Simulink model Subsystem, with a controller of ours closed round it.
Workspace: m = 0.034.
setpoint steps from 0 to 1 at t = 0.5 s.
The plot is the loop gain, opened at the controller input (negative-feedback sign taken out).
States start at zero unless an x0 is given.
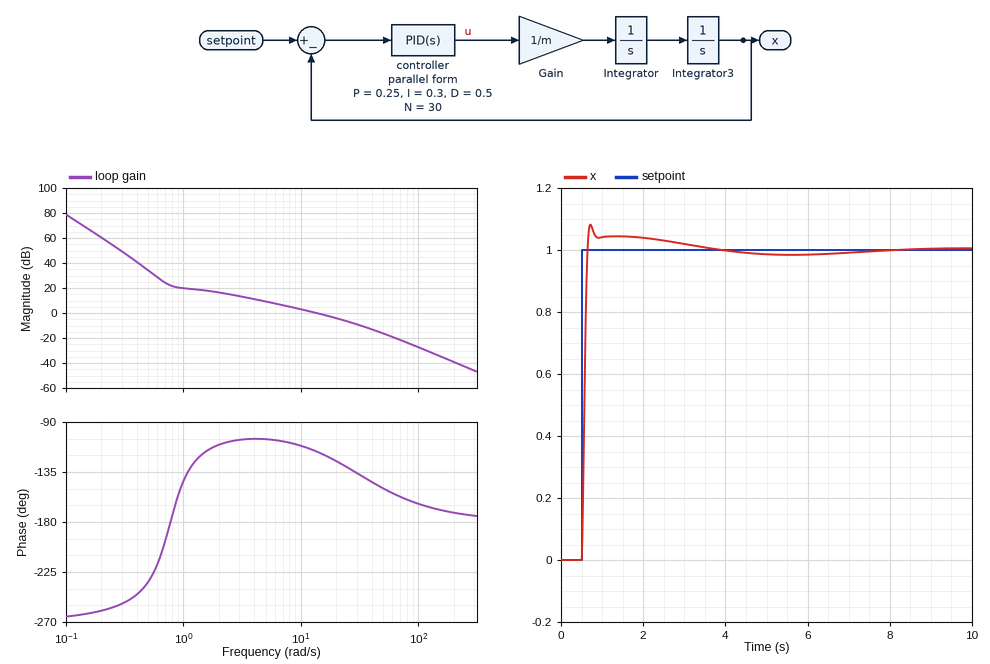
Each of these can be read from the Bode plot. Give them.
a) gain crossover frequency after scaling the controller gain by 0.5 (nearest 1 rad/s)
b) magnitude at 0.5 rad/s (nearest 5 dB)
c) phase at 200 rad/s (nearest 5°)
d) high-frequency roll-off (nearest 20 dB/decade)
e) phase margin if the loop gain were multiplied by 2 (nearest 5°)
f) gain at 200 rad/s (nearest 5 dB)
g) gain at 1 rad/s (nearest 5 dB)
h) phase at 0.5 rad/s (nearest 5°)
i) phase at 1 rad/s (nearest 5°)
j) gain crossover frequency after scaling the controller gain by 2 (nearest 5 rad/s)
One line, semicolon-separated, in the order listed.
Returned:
7 rad/s; 35 dB; -170°; -40 dB/decade; 50°; -40 dB; 20 dB; -235°; -145°; 25 rad/s
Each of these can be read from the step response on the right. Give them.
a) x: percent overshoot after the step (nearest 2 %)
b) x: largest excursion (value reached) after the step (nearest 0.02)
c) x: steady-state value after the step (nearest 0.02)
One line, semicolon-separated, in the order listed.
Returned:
8 %; 1.08; 1.00
